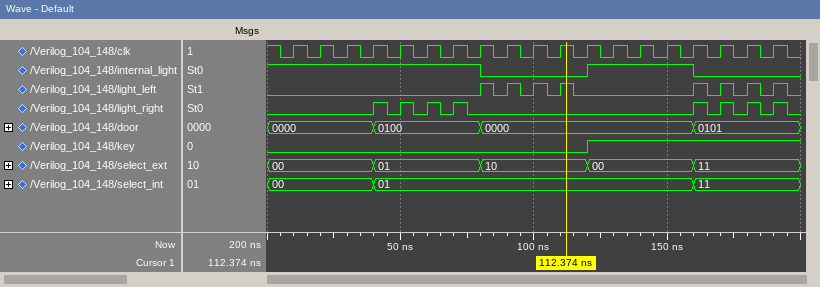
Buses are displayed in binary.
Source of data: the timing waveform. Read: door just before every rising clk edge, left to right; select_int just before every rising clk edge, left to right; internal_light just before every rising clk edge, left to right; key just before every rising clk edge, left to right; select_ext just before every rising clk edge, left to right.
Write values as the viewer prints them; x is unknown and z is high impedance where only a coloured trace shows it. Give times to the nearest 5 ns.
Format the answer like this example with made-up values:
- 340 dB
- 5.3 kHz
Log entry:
- 0000, 0000, 0000, 0000, 0100, 0100, 0100, 0100, 0000, 0000, 0000, 0000, 0000, 0000, 0000, 0000, 0101, 0101, 0101
- 00, 00, 00, 00, 01, 01, 01, 01, 01, 01, 01, 01, 01, 01, 01, 01, 11, 11, 11
- 1 1 1 1 1 1 1 1 0 0 0 0 1 1 1 1 0 0 0
- 0 0 0 0 0 0 0 0 0 0 0 0 1 1 1 1 1 1 1
- 00, 00, 00, 00, 01, 01, 01, 01, 10, 10, 10, 10, 00, 00, 00, 00, 11, 11, 11
